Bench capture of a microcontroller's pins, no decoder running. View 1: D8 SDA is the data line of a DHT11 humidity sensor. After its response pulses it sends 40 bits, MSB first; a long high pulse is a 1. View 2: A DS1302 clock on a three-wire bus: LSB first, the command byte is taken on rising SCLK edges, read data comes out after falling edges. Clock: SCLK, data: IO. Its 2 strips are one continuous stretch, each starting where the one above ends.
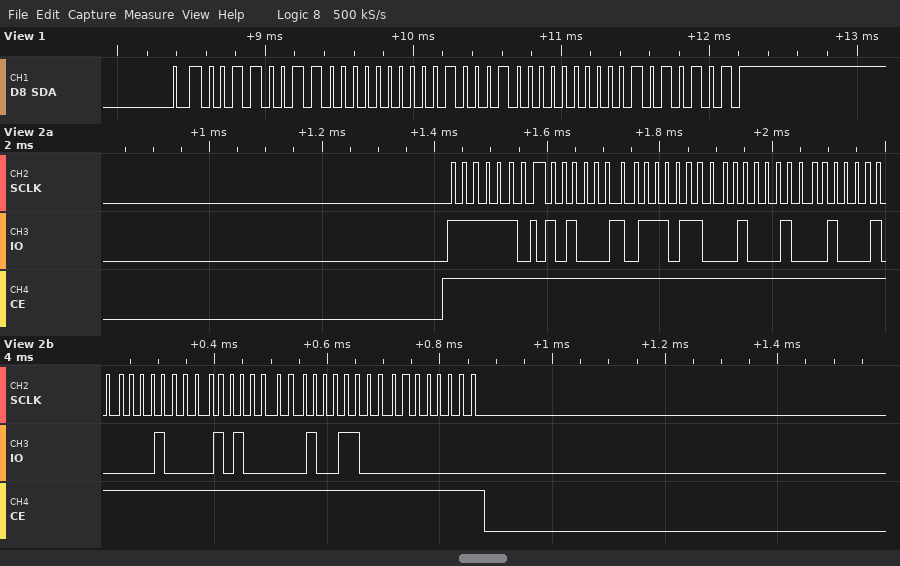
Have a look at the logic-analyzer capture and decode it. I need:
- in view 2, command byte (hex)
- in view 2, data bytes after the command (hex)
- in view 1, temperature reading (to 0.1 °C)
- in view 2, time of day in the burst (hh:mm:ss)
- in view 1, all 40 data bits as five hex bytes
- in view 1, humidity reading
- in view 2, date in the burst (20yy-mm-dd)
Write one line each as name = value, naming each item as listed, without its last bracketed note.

in view 2, command byte = 0xBF
in view 2, data bytes after the command = 45 37 22 22 08 05 19 00
in view 1, temperature reading = 34.0 °C
in view 2, time of day in the burst = 22:37:45
in view 1, all 40 data bits as five hex bytes = 33 00 22 00 55
in view 1, humidity reading = 51 %
in view 2, date in the burst = 2019-08-22
